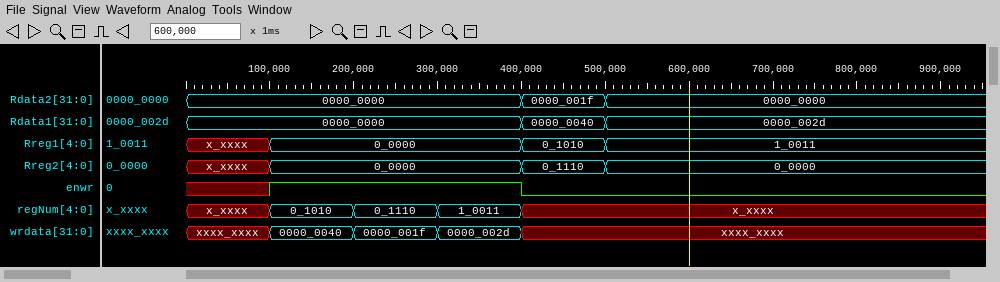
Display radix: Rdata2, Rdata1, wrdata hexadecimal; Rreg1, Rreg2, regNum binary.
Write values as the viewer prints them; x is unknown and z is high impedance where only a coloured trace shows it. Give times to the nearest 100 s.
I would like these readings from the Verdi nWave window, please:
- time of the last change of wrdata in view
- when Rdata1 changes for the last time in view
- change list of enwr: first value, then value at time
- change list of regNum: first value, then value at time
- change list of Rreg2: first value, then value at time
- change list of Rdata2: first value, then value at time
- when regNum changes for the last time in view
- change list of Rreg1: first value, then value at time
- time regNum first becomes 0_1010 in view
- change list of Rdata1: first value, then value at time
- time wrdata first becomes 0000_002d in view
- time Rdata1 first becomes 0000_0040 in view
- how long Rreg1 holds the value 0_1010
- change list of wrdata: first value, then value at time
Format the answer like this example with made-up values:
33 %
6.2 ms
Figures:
400 s
500 s
x, 1 at 100 s, 0 at 400 s
x_xxxx, 0_1010 at 100 s, 0_1110 at 200 s, 1_0011 at 300 s, x_xxxx at 400 s
x_xxxx, 0_0000 at 100 s, 0_1110 at 400 s, 0_0000 at 500 s
0000_0000, 0000_001f at 400 s, 0000_0000 at 500 s
400 s
x_xxxx, 0_0000 at 100 s, 0_1010 at 400 s, 1_0011 at 500 s
100 s
0000_0000, 0000_0040 at 400 s, 0000_002d at 500 s
300 s
400 s
100 s
xxxx_xxxx, 0000_0040 at 100 s, 0000_001f at 200 s, 0000_002d at 300 s, xxxx_xxxx at 400 s
